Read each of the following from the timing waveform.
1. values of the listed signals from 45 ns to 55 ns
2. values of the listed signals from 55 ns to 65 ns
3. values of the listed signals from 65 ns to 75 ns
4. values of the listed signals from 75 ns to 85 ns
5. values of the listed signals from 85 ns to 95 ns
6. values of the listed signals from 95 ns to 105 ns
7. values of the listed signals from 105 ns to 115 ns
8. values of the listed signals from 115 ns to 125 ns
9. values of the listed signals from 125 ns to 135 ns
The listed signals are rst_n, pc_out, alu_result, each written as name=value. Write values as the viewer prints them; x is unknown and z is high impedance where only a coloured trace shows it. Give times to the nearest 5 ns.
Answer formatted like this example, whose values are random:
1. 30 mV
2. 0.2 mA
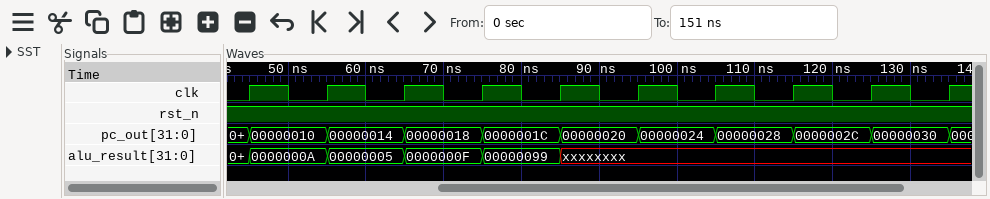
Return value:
1. rst_n=1, pc_out=00000010, alu_result=0000000A
2. rst_n=1, pc_out=00000014, alu_result=00000005
3. rst_n=1, pc_out=00000018, alu_result=0000000F
4. rst_n=1, pc_out=0000001C, alu_result=00000099
5. rst_n=1, pc_out=00000020, alu_result=xxxxxxxx
6. rst_n=1, pc_out=00000024, alu_result=xxxxxxxx
7. rst_n=1, pc_out=00000028, alu_result=xxxxxxxx
8. rst_n=1, pc_out=0000002C, alu_result=xxxxxxxx
9. rst_n=1, pc_out=00000030, alu_result=xxxxxxxx
